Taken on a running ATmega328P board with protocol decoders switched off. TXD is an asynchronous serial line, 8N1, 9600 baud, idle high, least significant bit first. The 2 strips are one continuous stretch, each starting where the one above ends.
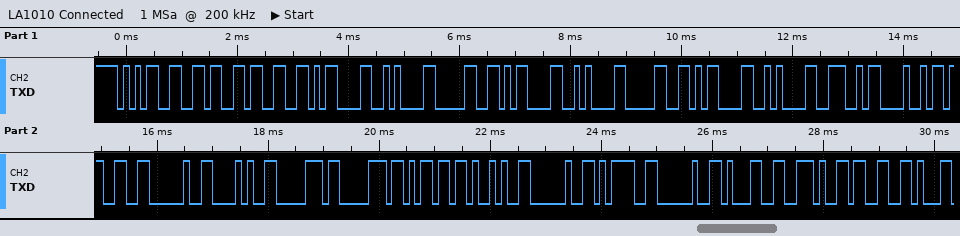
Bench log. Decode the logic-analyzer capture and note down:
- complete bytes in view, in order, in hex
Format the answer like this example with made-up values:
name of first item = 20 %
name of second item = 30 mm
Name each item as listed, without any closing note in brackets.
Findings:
complete bytes in view, in order, in hex = 0x35 0x36 0x33 0x0D 0x0A 0x30 0x0D 0x0A 0x30 0x0D 0x0A 0x4E 0x48 0x33 0x20 0x28 0x70 0x70 0x6D 0x29 0x20 0x3D 0x20 0x31 0x2E 0x33
